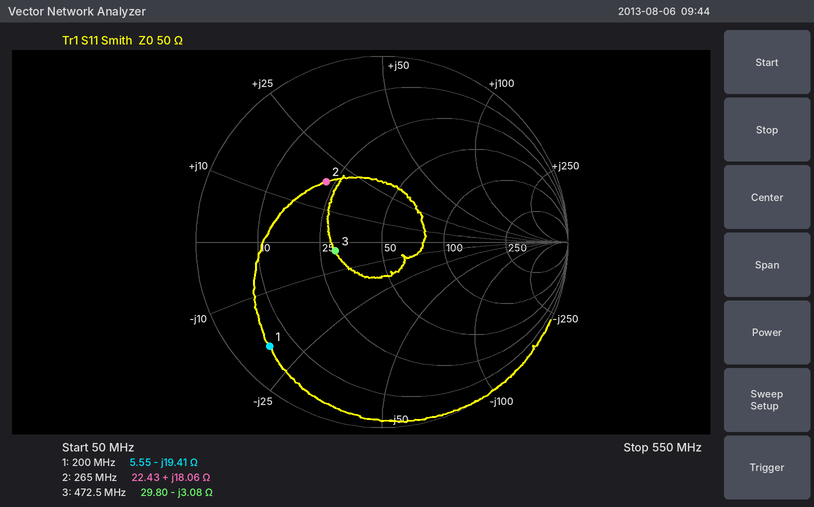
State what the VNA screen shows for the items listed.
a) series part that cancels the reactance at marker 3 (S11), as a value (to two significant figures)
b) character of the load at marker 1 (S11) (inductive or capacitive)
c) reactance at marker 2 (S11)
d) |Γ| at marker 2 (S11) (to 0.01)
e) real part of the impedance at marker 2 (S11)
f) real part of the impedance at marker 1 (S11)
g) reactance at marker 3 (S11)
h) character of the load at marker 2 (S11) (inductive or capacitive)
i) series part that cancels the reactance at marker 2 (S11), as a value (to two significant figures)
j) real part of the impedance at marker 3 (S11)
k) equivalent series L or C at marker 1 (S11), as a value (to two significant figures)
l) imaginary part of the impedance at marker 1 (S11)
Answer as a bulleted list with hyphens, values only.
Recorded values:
- 1.0 nH
- capacitive
- +18.06 Ω
- 0.44
- 22.43 Ω
- 5.55 Ω
- -3.08 Ω
- inductive
- 33 pF
- 29.80 Ω
- 41 pF
- -19.41 Ω
